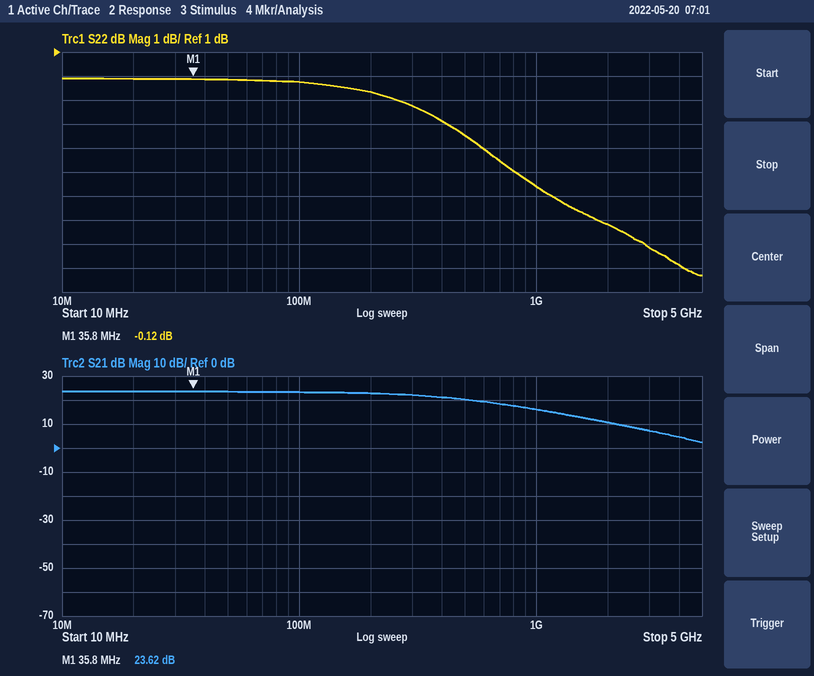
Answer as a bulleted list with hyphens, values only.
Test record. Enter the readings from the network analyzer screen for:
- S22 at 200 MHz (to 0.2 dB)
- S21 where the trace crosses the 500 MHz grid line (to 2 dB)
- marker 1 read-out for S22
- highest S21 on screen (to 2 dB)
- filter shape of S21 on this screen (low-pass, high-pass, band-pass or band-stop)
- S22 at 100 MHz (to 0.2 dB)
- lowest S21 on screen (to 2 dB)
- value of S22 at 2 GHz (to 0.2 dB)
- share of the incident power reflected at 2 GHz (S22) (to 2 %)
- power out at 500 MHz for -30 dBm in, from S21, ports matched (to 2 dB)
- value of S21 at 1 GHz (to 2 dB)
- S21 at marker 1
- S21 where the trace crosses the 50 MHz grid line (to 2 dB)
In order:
- -0.6 dB
- 20 dB
- -0.12 dB
- 24 dB
- low-pass
- -0.2 dB
- 2 dB
- -6.2 dB
- 24 %
- -10 dBm
- 16 dB
- 23.62 dB
- 24 dB
